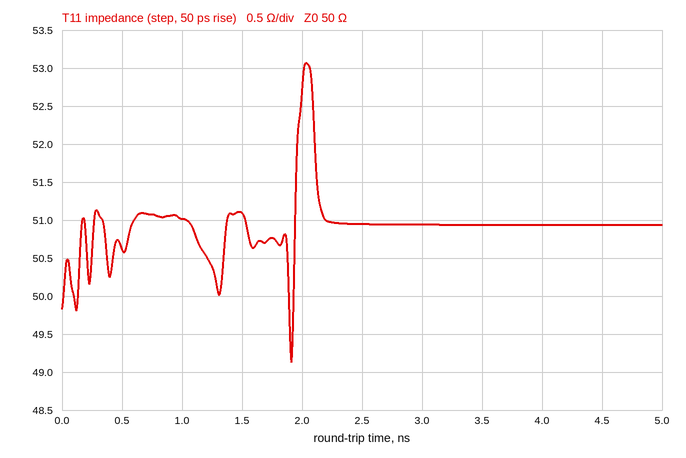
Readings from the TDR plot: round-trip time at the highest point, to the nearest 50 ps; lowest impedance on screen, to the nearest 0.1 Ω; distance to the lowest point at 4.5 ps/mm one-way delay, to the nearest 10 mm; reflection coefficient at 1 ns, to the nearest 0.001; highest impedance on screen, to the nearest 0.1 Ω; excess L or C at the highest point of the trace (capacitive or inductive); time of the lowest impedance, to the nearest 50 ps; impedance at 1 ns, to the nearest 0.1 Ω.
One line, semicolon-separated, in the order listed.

2.05 ns; 49.1 Ω; 210 mm; +0.010; 53.1 Ω; inductive; 1.90 ns; 51.0 Ω
